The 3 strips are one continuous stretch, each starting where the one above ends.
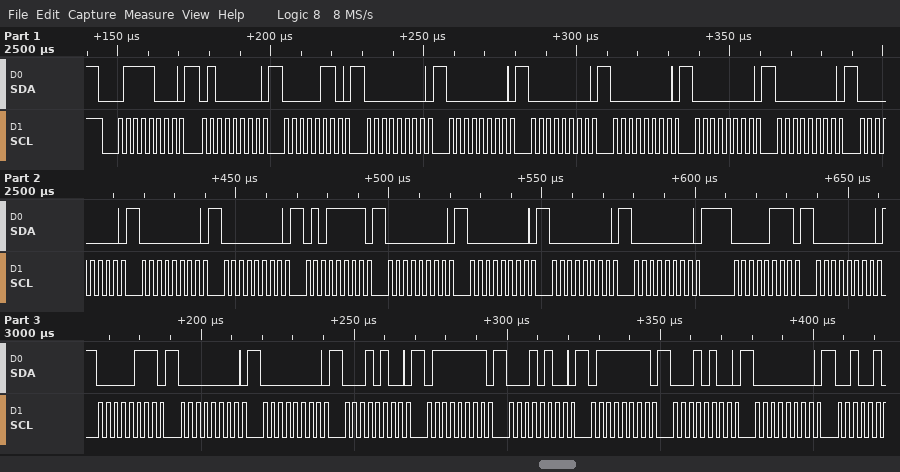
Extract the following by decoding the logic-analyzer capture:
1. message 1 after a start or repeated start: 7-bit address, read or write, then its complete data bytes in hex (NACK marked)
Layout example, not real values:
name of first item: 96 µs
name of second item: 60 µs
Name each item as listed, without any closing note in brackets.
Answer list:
message 1 after a start or repeated start: 7-bit address, read or write, then its complete data bytes in hex: 0x3C write: 40 06 00 00 00 00 00 00 00 00 00 5F 00 00 00 00 07 00 07 00 00 14 7F 14 7F 14 00
